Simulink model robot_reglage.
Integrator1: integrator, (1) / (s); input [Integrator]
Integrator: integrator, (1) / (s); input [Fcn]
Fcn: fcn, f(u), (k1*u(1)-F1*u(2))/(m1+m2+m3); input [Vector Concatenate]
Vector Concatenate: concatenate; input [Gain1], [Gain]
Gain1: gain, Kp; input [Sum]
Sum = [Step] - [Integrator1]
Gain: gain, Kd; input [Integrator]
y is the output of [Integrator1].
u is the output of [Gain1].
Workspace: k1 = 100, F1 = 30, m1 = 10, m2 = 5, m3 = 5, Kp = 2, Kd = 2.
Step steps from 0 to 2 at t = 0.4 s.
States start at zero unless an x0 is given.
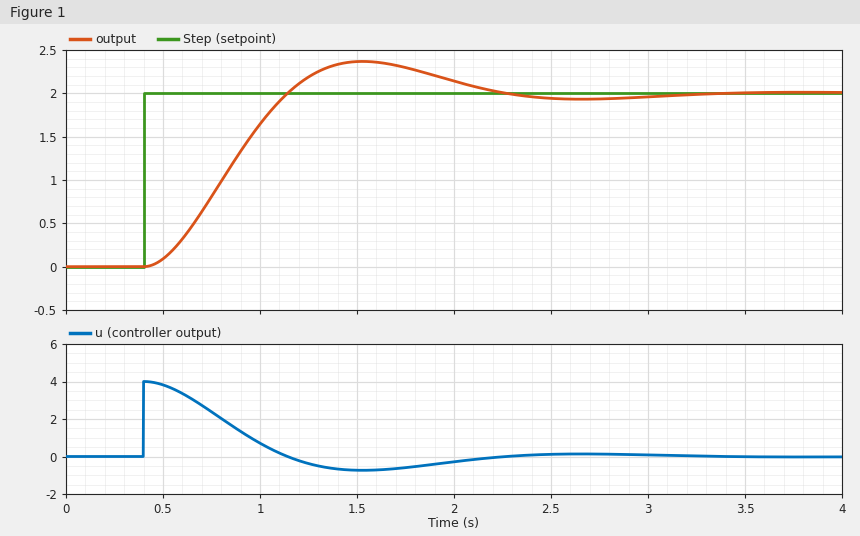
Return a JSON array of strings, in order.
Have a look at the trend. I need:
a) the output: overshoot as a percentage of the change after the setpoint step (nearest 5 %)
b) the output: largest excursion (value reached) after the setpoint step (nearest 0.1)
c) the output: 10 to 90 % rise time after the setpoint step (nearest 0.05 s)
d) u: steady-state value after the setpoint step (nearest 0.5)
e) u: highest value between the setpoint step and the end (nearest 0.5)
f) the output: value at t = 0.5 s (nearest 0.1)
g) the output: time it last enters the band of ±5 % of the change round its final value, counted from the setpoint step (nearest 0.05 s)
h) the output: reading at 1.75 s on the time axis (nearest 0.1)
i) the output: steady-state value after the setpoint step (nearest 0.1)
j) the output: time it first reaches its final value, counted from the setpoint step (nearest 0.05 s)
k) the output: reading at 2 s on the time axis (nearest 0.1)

["20 %", "2.4", "0.50 s", "0.0", "4.0", "0.1", "1.65 s", "2.3", "2.0", "0.75 s", "2.1"]
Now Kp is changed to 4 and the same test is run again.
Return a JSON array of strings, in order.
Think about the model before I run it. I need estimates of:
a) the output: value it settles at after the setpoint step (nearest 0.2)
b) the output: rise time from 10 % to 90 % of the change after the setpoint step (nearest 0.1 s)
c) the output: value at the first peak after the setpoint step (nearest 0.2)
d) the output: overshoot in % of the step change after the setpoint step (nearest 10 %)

["2.0", "0.3 s", "2.6", "30 %"]
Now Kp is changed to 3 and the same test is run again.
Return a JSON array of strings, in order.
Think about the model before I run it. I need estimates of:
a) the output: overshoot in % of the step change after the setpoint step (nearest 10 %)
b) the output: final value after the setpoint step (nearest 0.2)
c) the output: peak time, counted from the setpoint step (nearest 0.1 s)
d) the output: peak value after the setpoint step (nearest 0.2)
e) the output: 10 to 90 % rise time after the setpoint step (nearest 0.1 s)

["30 %", "2.0", "0.9 s", "2.6", "0.4 s"]
